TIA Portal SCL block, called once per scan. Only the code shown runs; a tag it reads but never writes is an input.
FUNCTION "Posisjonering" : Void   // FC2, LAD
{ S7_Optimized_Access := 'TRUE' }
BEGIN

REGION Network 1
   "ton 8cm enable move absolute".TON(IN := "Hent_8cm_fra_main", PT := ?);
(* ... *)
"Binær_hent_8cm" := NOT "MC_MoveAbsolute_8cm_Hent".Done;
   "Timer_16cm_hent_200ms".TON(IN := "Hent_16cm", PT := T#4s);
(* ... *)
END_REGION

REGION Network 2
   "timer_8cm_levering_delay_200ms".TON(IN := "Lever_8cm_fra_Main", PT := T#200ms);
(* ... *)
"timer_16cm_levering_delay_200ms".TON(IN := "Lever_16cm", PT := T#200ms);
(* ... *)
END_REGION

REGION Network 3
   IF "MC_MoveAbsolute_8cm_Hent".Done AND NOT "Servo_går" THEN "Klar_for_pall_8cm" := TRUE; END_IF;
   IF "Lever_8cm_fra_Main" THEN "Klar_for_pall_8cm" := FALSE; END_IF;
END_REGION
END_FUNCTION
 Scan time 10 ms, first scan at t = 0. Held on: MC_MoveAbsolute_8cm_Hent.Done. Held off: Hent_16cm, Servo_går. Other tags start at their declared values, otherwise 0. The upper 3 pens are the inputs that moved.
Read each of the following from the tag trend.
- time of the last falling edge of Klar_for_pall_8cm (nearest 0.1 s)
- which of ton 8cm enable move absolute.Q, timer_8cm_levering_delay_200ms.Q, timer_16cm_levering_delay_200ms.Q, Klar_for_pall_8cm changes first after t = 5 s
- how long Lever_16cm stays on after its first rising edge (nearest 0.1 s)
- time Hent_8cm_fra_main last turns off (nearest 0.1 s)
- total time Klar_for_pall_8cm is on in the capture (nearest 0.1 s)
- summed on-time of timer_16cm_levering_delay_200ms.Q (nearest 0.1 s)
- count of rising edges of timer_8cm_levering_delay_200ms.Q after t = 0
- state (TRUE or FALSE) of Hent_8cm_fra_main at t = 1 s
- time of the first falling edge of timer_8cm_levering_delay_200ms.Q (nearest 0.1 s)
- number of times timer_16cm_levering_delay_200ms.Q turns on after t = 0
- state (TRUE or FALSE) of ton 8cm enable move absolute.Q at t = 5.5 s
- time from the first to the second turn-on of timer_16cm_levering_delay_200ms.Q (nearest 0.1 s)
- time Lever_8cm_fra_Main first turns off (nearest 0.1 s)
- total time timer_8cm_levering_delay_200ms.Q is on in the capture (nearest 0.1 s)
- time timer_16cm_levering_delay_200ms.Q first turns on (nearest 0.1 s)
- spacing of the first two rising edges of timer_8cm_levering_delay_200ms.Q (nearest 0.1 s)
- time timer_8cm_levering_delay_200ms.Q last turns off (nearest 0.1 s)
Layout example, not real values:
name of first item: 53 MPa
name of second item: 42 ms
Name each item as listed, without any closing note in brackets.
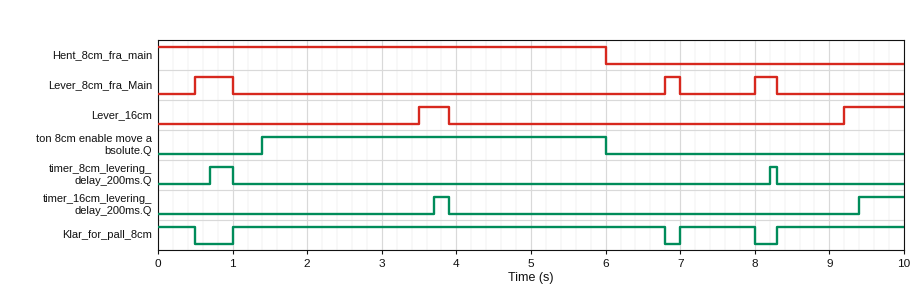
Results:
time of the last falling edge of Klar_for_pall_8cm: 8.0 s
which of ton 8cm enable move absolute.Q, timer_8cm_levering_delay_200ms.Q, timer_16cm_levering_delay_200ms.Q, Klar_for_pall_8cm changes first after t = 5 s: ton 8cm enable move absolute.Q
how long Lever_16cm stays on after its first rising edge: 0.4 s
time Hent_8cm_fra_main last turns off: 6.0 s
total time Klar_for_pall_8cm is on in the capture: 9.0 s
summed on-time of timer_16cm_levering_delay_200ms.Q: 0.8 s
count of rising edges of timer_8cm_levering_delay_200ms.Q after t = 0: 2
state (TRUE or FALSE) of Hent_8cm_fra_main at t = 1 s: TRUE
time of the first falling edge of timer_8cm_levering_delay_200ms.Q: 1.0 s
number of times timer_16cm_levering_delay_200ms.Q turns on after t = 0: 2
state (TRUE or FALSE) of ton 8cm enable move absolute.Q at t = 5.5 s: TRUE
time from the first to the second turn-on of timer_16cm_levering_delay_200ms.Q: 5.7 s
time Lever_8cm_fra_Main first turns off: 1.0 s
total time timer_8cm_levering_delay_200ms.Q is on in the capture: 0.4 s
time timer_16cm_levering_delay_200ms.Q first turns on: 3.7 s
spacing of the first two rising edges of timer_8cm_levering_delay_200ms.Q: 7.5 s
time timer_8cm_levering_delay_200ms.Q last turns off: 8.3 s
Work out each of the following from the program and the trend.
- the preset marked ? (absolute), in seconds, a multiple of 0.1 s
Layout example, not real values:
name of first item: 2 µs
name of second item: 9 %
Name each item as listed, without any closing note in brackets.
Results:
the preset marked ? (absolute), in seconds, a multiple of 0.1 s: 1.4 s
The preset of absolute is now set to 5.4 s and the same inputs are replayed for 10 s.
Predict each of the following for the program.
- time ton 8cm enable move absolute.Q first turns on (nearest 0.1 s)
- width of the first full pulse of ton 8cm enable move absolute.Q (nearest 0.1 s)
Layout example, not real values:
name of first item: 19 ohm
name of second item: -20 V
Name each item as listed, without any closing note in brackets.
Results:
time ton 8cm enable move absolute.Q first turns on: 5.4 s
width of the first full pulse of ton 8cm enable move absolute.Q: 0.6 s
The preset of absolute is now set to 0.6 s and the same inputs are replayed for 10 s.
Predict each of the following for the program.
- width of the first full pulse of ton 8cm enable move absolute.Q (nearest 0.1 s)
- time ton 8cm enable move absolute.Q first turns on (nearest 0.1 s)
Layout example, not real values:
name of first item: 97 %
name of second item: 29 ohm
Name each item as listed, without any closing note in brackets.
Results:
width of the first full pulse of ton 8cm enable move absolute.Q: 5.4 s
time ton 8cm enable move absolute.Q first turns on: 0.6 s
